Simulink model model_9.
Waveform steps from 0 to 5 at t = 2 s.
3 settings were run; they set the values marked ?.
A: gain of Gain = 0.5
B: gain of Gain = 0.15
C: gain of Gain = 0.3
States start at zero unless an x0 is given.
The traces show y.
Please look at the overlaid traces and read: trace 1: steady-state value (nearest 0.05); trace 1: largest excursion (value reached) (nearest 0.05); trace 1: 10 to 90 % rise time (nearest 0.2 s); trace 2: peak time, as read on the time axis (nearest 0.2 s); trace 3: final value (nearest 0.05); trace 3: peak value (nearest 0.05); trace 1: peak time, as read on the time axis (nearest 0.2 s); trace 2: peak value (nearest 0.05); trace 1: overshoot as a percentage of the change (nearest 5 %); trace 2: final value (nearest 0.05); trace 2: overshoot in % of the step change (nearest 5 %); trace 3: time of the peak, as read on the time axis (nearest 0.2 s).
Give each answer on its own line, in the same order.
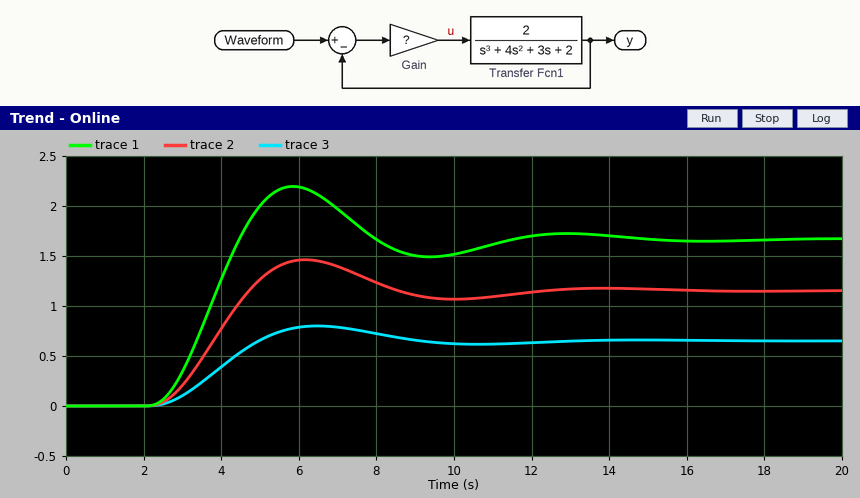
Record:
1.65
2.20
1.6 s
6.2 s
0.65
0.80
5.8 s
1.45
30 %
1.15
25 %
6.4 s
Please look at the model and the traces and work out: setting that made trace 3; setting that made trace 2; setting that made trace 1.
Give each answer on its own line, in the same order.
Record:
B
C
A
